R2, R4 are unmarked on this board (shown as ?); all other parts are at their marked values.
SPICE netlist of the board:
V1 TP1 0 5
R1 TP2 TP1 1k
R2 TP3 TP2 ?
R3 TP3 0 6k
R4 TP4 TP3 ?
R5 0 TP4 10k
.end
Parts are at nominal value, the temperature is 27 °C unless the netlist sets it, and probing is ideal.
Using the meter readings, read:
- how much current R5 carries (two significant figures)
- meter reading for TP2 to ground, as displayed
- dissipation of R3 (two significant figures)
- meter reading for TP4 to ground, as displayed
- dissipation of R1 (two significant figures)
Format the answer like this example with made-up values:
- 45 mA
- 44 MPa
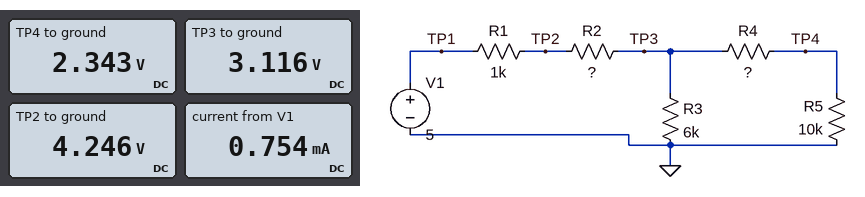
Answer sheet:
- 230 µA
- 4.246 V
- 1.6 mW
- 2.343 V
- 570 µW
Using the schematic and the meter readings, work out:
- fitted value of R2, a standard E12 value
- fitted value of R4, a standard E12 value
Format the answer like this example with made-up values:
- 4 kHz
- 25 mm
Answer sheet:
- 1.5 kΩ
- 3.3 kΩ
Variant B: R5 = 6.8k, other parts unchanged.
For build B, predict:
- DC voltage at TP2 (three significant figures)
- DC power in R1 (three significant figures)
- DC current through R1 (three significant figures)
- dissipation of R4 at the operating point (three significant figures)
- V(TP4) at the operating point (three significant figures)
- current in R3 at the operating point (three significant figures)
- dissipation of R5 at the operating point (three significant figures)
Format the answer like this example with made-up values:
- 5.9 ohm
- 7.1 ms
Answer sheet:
- 4.20 V
- 637 µW
- 798 µA
- 292 µW
- 2.02 V
- 501 µA
- 602 µW
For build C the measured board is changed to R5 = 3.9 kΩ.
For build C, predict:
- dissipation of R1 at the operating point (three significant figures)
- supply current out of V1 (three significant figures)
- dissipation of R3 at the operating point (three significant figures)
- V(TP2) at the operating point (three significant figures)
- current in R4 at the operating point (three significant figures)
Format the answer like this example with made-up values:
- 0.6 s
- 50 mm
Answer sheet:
- 750 µW
- 866 µA
- 1.34 mW
- 4.13 V
- 394 µA
